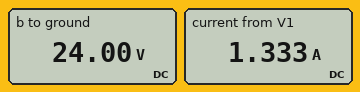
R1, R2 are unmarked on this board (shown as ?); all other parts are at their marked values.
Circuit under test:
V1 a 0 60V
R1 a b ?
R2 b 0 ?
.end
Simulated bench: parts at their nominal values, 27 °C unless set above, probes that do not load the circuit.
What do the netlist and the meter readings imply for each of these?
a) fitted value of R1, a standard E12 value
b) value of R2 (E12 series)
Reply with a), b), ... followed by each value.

a) 27 Ω
b) 18 Ω
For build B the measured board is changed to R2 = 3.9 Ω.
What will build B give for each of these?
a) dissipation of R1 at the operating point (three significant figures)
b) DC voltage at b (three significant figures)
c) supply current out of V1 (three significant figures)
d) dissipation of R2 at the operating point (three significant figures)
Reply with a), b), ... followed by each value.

a) 102 W
b) 7.57 V
c) 1.94 A
d) 14.7 W
